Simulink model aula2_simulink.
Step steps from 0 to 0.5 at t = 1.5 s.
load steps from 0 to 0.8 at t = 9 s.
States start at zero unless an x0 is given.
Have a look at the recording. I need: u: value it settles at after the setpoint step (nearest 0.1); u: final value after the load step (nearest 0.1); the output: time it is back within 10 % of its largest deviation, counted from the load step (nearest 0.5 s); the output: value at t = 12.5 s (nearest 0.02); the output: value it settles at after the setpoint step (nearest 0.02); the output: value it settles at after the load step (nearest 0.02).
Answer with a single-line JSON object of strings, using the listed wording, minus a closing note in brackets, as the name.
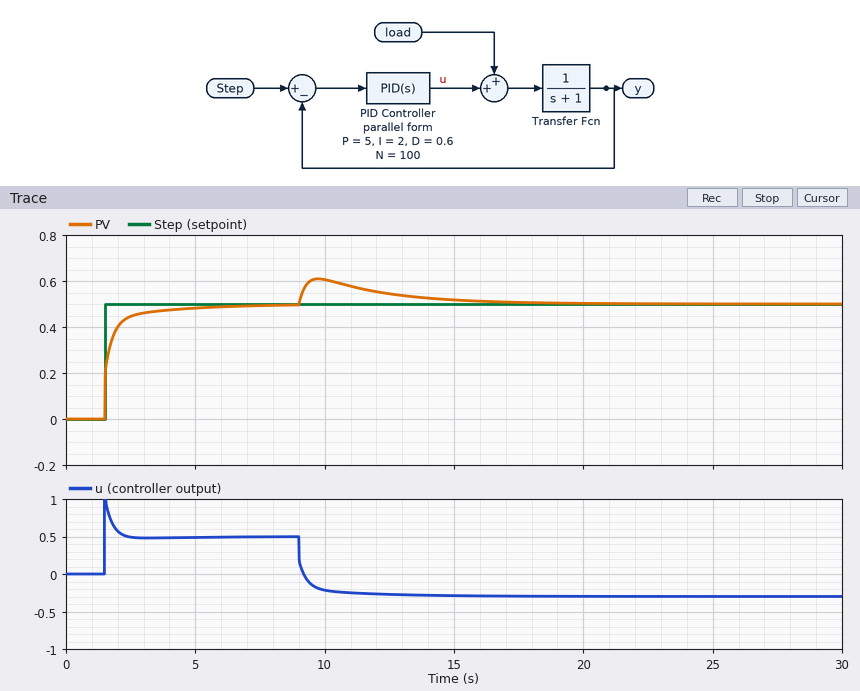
{"u: value it settles at after the setpoint step": "0.5", "u: final value after the load step": "-0.3", "the output: time it is back within 10 % of its largest deviation, counted from the load step": "7.0 s", "the output: value at t = 12.5 s": "0.54", "the output: value it settles at after the setpoint step": "0.50", "the output: value it settles at after the load step": "0.50"}
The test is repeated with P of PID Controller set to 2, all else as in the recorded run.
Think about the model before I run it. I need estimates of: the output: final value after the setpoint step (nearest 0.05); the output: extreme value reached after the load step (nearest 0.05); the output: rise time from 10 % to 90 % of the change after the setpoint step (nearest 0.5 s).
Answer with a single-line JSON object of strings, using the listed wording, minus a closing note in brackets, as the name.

{"the output: final value after the setpoint step": "0.50", "the output: extreme value reached after the load step": "0.70", "the output: rise time from 10 % to 90 % of the change after the setpoint step": "1.5 s"}
